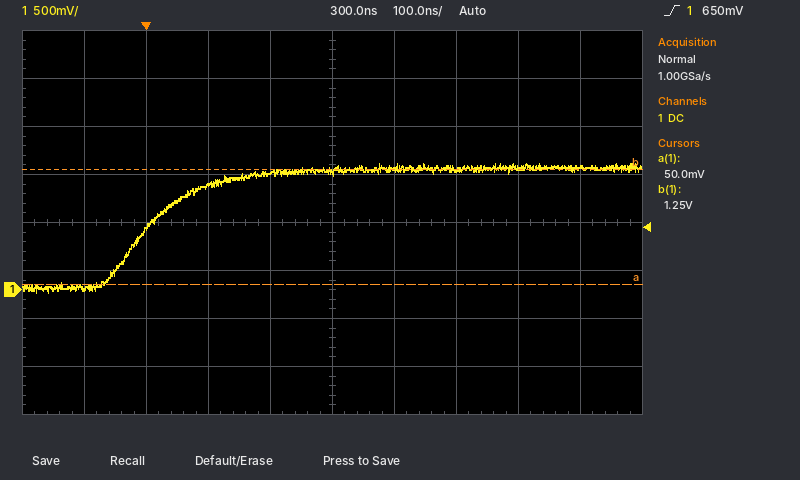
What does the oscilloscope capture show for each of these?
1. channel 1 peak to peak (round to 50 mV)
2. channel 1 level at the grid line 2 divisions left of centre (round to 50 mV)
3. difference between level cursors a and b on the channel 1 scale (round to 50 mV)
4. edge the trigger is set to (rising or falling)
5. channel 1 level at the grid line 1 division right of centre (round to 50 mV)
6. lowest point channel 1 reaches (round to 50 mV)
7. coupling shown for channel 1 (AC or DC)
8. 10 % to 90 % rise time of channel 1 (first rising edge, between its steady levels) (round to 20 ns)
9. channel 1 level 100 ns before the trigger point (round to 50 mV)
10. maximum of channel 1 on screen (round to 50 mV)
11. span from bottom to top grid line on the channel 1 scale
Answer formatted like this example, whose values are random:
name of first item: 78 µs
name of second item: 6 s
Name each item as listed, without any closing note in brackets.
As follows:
channel 1 peak to peak: 1.35 V
channel 1 level at the grid line 2 divisions left of centre: 1.10 V
difference between level cursors a and b on the channel 1 scale: 1.20 V
edge the trigger is set to: rising
channel 1 level at the grid line 1 division right of centre: 1.25 V
lowest point channel 1 reaches: -50 mV
coupling shown for channel 1: DC
10 % to 90 % rise time of channel 1 (first rising edge, between its steady levels): 180 ns
channel 1 level 100 ns before the trigger point: 0 mV
maximum of channel 1 on screen: 1.30 V
span from bottom to top grid line on the channel 1 scale: 4 V
